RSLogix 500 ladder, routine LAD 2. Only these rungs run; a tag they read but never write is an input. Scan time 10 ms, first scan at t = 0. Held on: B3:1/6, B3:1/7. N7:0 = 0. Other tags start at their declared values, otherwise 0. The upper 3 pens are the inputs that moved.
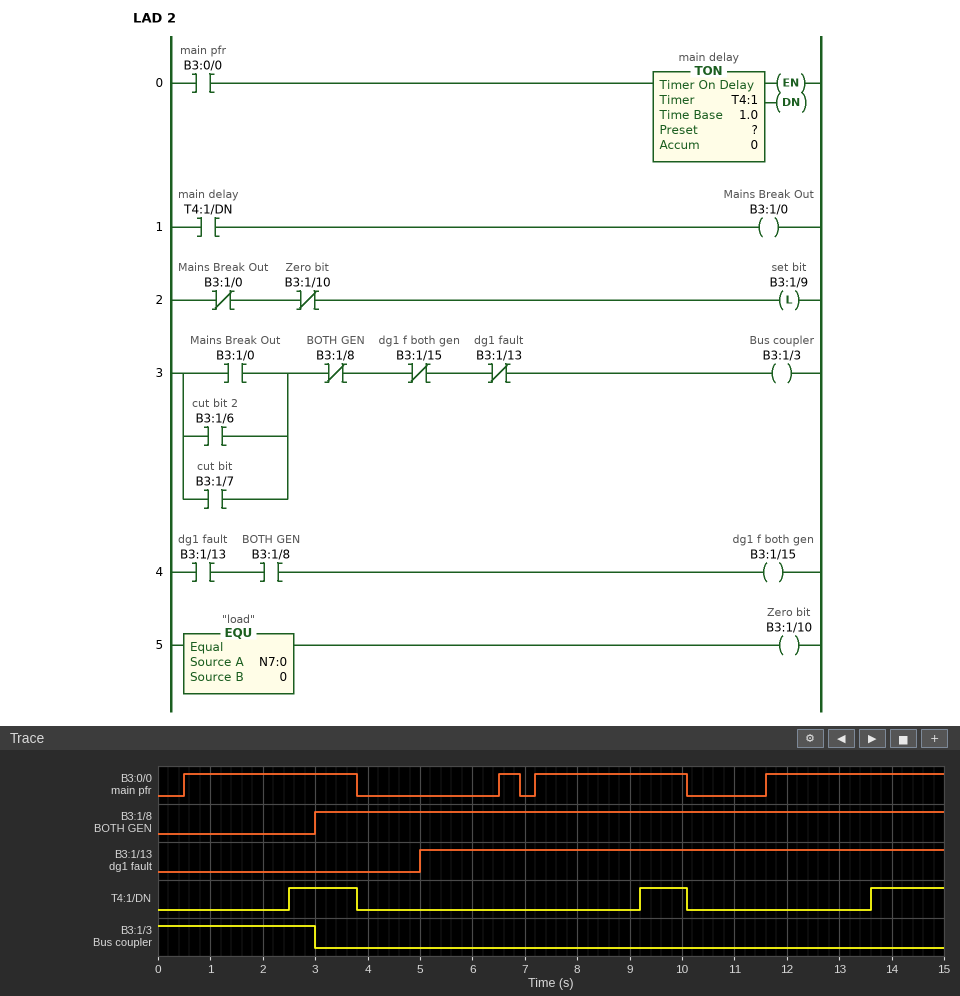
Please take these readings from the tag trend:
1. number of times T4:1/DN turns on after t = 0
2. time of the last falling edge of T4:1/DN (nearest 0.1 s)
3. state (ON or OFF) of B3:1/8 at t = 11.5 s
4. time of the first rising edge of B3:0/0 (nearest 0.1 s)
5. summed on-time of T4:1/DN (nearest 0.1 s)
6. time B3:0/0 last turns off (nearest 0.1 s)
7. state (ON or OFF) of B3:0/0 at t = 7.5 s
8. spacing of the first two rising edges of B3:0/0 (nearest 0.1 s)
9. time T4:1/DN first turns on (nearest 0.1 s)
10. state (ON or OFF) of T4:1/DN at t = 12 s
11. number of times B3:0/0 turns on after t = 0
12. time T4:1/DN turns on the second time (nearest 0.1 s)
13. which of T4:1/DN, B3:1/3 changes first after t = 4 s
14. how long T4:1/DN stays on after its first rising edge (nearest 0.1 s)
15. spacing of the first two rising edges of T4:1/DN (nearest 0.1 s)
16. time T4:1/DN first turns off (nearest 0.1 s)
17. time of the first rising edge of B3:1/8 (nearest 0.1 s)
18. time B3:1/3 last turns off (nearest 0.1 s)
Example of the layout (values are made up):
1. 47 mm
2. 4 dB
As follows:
1. 3
2. 10.1 s
3. ON
4. 0.5 s
5. 3.6 s
6. 10.1 s
7. ON
8. 6.0 s
9. 2.5 s
10. OFF
11. 4
12. 9.2 s
13. T4:1/DN
14. 1.3 s
15. 6.7 s
16. 3.8 s
17. 3.0 s
18. 3.0 s
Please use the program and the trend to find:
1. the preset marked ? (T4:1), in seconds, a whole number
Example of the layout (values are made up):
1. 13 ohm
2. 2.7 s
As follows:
1. 2 s
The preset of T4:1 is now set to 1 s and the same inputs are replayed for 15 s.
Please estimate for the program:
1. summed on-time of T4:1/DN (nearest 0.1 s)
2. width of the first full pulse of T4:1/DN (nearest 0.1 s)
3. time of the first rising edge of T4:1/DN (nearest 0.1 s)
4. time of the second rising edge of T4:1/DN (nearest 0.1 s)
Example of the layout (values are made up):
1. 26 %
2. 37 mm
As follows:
1. 6.6 s
2. 2.3 s
3. 1.5 s
4. 8.2 s
